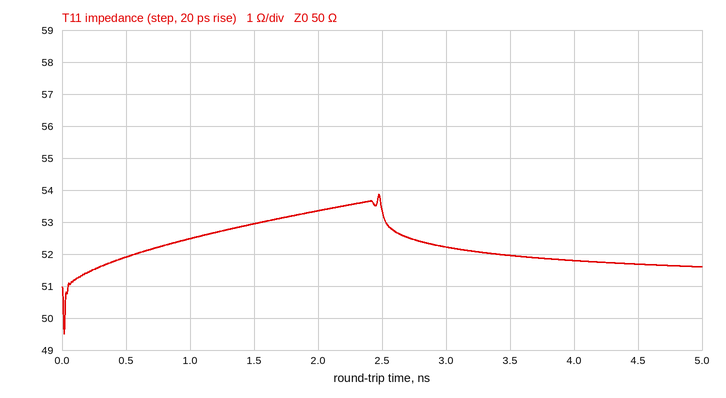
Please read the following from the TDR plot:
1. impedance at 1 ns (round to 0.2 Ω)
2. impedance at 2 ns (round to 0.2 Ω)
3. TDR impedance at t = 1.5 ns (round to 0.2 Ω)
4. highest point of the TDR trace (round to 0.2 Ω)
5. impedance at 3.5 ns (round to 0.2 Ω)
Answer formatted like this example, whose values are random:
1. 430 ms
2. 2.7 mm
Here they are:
1. 52.4 Ω
2. 53.4 Ω
3. 53.0 Ω
4. 53.8 Ω
5. 52.0 Ω
